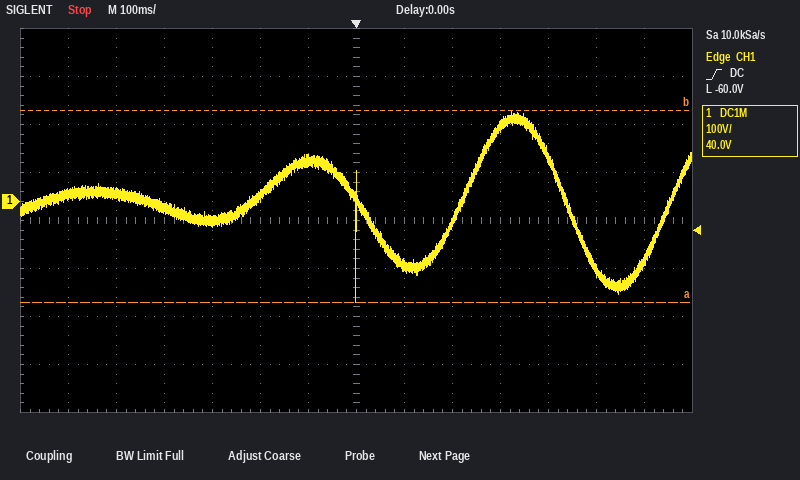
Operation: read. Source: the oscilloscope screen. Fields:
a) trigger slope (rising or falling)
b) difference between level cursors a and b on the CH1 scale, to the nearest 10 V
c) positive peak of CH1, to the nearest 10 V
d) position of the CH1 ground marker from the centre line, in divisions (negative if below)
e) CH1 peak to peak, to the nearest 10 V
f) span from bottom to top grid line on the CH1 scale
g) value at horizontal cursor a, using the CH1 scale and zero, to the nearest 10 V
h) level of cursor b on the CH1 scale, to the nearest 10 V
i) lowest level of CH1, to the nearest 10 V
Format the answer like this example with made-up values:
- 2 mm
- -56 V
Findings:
- rising
- 400 V
- 190 V
- +0.4 div
- 400 V
- 800 V
- -210 V
- 190 V
- -210 V
